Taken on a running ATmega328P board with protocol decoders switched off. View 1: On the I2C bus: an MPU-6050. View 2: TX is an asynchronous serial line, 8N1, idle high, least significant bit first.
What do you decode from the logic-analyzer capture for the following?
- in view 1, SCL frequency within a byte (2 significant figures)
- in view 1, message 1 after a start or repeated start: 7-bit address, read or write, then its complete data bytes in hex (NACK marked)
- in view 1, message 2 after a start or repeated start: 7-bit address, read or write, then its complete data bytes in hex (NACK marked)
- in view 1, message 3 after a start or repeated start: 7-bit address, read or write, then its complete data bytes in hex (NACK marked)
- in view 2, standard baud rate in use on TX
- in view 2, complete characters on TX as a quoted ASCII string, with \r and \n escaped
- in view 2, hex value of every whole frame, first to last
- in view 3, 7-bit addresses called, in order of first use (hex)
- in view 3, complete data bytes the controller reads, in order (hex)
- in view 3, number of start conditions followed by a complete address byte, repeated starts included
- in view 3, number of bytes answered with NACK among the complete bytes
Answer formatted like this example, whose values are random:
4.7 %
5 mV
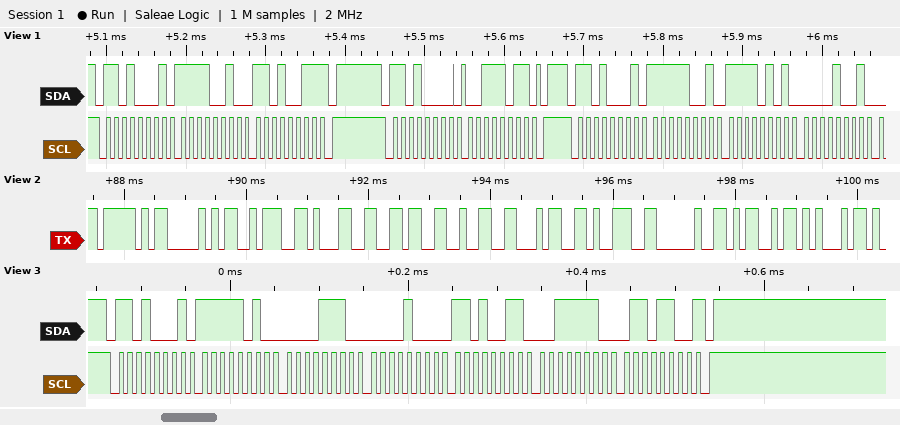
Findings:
100 kHz
0x68 read: F2 D3 NACK
0x68 write: 3B
0x68 read: F9 F5 09
9600 baud
"_P:16249 ME"
5F 50 3A 31 36 32 34 39 20 4D 45
0x68
FA 0E 08 D3 3E 6C
1
1
